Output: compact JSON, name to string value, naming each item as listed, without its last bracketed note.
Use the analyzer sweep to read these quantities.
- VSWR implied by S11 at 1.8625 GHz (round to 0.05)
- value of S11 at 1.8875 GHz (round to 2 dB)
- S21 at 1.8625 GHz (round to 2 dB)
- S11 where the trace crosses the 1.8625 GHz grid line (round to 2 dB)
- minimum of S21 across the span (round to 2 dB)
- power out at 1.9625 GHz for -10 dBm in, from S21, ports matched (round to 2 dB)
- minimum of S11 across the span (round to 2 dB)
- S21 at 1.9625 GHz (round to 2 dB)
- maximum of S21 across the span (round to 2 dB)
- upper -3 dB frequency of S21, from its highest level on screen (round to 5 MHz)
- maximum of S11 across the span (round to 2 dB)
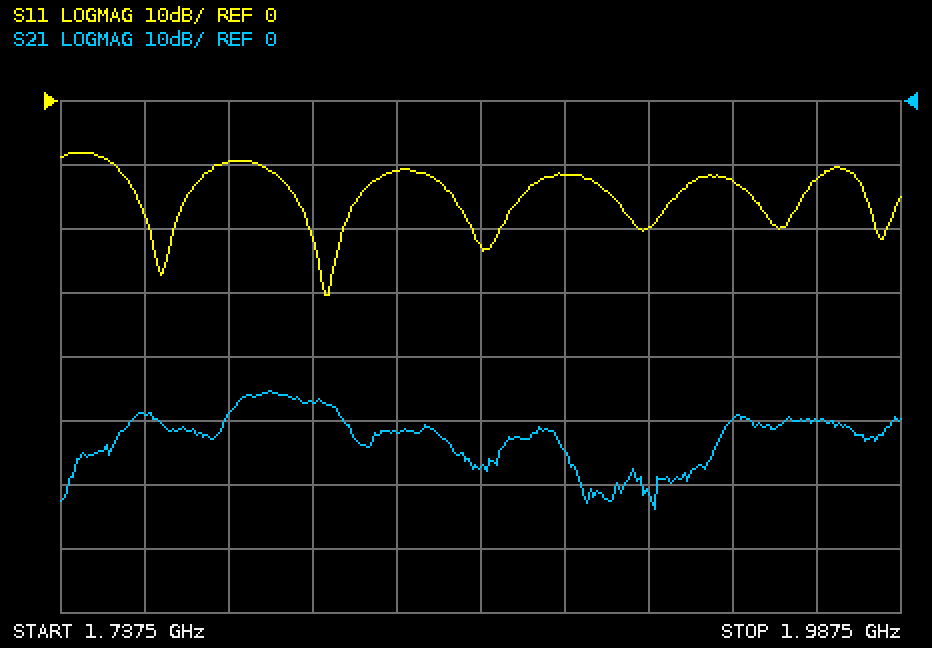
{"VSWR implied by S11 at 1.8625 GHz": "1.15", "value of S11 at 1.8875 GHz": "-12 dB", "S21 at 1.8625 GHz": "-58 dB", "S11 where the trace crosses the 1.8625 GHz grid line": "-22 dB", "minimum of S21 across the span": "-64 dB", "power out at 1.9625 GHz for -10 dBm in, from S21, ports matched": "-60 dBm", "minimum of S11 across the span": "-30 dB", "S21 at 1.9625 GHz": "-50 dB", "maximum of S21 across the span": "-46 dB", "upper -3 dB frequency of S21, from its highest level on screen": "1.820 GHz", "maximum of S11 across the span": "-8 dB"}
